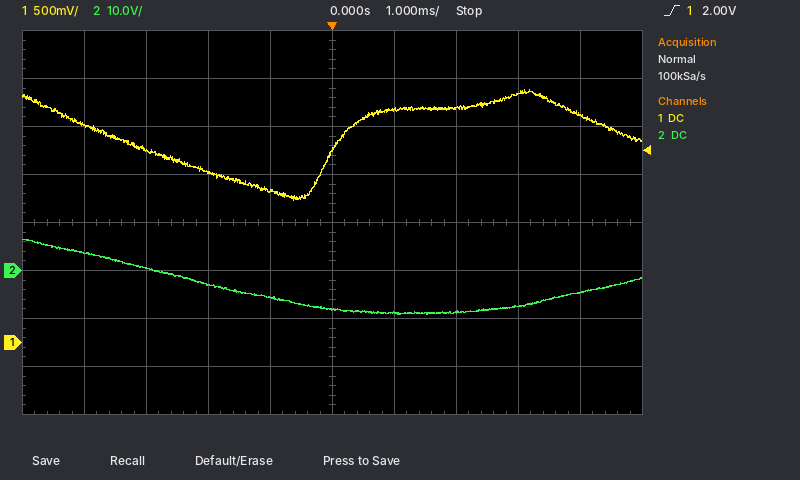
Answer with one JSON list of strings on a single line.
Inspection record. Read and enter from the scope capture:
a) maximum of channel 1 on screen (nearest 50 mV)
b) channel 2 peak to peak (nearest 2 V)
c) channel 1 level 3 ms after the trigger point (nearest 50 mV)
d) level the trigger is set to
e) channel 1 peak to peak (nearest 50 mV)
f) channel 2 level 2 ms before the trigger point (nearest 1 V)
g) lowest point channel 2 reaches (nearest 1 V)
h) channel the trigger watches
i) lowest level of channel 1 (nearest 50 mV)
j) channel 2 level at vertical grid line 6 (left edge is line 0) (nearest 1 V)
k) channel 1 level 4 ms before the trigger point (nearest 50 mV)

["2.65 V", "16 V", "2.60 V", "2.00 V", "1.15 V", "-3 V", "-9 V", "channel 1", "1.50 V", "-9 V", "2.25 V"]
